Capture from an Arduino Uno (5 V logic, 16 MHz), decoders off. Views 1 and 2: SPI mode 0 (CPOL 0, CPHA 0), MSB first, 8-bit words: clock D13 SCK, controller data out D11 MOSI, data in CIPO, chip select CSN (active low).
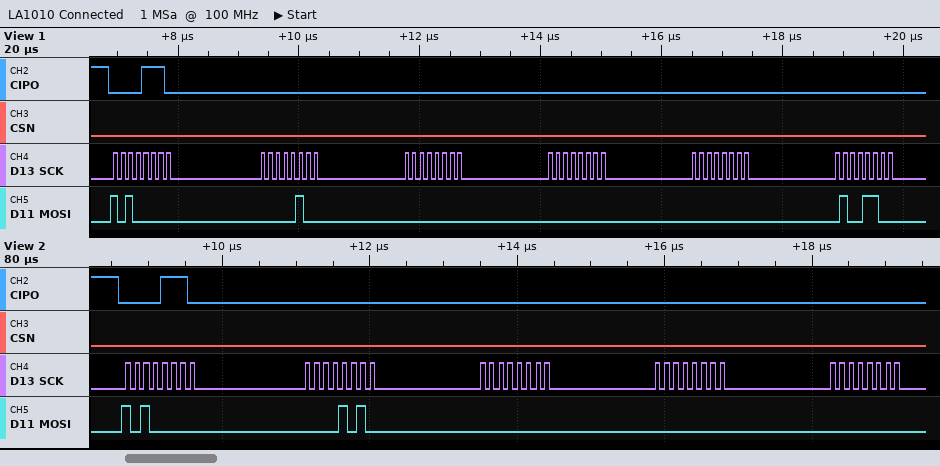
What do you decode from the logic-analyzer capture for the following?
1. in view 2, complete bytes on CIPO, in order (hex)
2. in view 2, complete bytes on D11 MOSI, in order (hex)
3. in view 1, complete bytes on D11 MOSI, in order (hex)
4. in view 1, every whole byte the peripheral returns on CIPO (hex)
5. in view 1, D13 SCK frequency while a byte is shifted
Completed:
0E 00 00 00 00
A0 0A 00 00 00
0xA0 0x04 0x00 0x00 0x00 0x4C
0x0E 0x00 0x00 0x00 0x00 0x00
8 MHz
